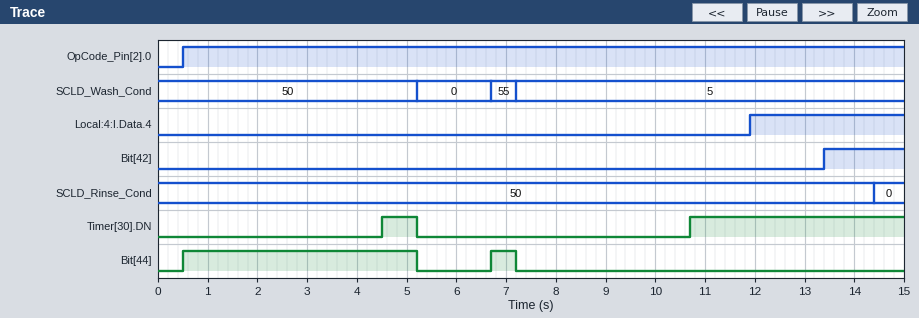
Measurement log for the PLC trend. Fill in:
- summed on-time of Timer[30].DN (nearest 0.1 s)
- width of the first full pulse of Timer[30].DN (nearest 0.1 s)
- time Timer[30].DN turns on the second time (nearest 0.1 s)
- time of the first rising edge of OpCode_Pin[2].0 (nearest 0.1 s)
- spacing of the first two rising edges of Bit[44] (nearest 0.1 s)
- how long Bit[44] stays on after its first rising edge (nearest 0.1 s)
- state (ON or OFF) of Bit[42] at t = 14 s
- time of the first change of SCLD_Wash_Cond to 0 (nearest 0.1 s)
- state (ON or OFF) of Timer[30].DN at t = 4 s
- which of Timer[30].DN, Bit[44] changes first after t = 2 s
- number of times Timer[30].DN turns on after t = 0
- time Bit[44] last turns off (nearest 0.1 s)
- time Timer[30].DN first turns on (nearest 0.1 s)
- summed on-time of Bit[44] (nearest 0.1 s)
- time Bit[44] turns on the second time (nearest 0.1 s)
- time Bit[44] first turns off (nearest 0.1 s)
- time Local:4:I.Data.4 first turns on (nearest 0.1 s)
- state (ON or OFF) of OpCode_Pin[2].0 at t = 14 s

5.0 s
0.7 s
10.7 s
0.5 s
6.2 s
4.7 s
ON
5.2 s
OFF
Timer[30].DN
2
7.2 s
4.5 s
5.2 s
6.7 s
5.2 s
11.9 s
ON
